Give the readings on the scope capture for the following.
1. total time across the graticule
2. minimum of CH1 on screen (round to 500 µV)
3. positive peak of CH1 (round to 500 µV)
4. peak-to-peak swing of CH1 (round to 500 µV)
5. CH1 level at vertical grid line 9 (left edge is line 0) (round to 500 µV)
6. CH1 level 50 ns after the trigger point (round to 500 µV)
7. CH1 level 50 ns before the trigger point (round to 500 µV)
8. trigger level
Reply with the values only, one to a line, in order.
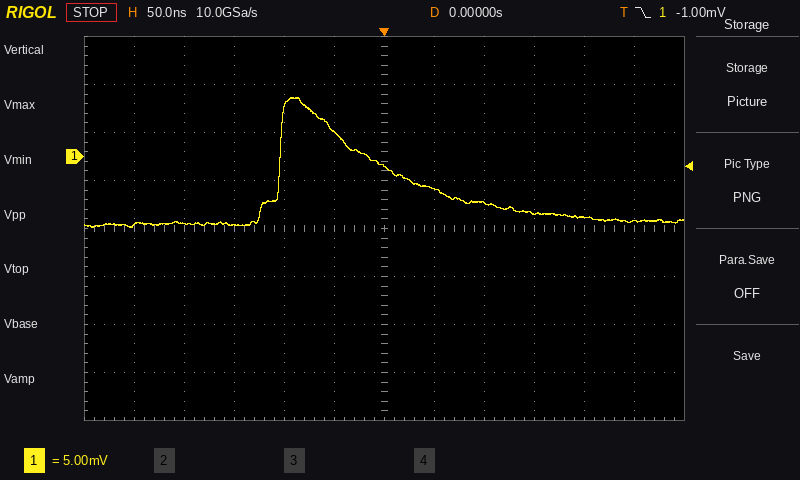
600 ns
-7.5 mV
6.0 mV
13.5 mV
-6.0 mV
-3.5 mV
2.5 mV
-1.00 mV
